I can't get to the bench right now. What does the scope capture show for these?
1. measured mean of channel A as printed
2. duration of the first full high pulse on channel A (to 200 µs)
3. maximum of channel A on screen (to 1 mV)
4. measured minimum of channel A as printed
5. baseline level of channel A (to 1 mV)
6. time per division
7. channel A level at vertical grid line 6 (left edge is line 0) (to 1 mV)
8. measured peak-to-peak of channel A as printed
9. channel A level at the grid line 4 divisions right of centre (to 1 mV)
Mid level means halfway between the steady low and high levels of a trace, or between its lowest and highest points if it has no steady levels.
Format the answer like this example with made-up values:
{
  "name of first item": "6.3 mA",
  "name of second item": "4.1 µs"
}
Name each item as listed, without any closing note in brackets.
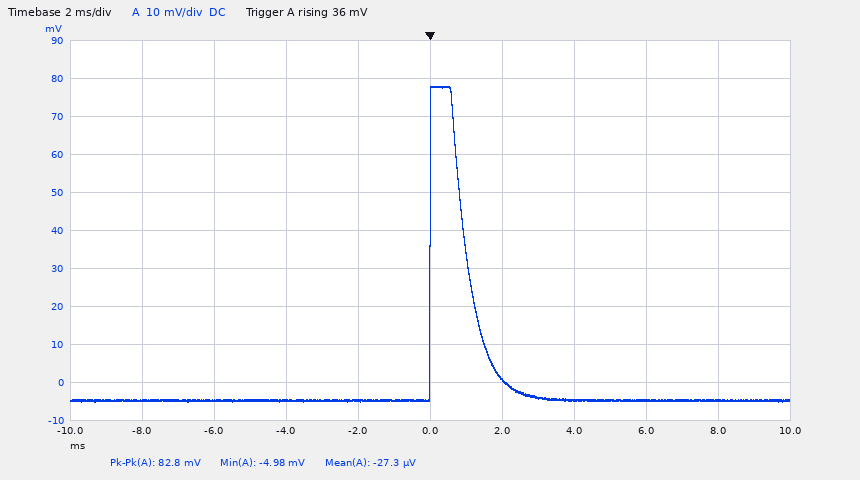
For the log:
{
  "measured mean of channel A as printed": "-27.3 µV",
  "duration of the first full high pulse on channel A": "1.0 ms",
  "maximum of channel A on screen": "78 mV",
  "measured minimum of channel A as printed": "-4.98 mV",
  "baseline level of channel A": "-5 mV",
  "time per division": "2 ms",
  "channel A level at vertical grid line 6 (left edge is line 0)": "1 mV",
  "measured peak-to-peak of channel A as printed": "82.8 mV",
  "channel A level at the grid line 4 divisions right of centre": "-5 mV"
}
